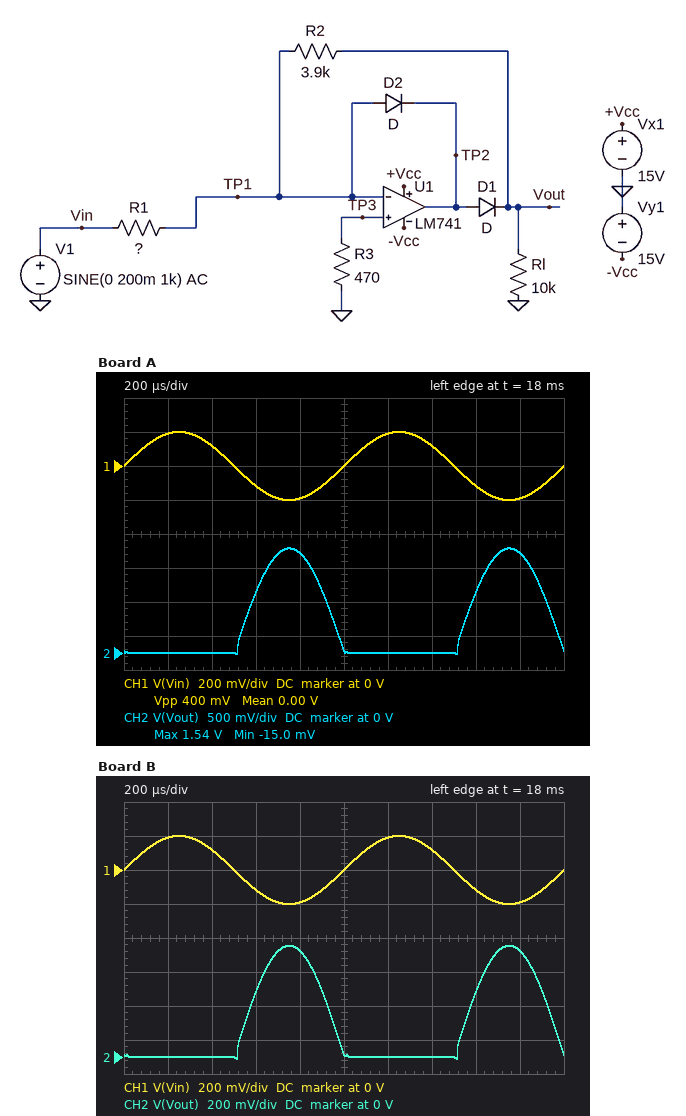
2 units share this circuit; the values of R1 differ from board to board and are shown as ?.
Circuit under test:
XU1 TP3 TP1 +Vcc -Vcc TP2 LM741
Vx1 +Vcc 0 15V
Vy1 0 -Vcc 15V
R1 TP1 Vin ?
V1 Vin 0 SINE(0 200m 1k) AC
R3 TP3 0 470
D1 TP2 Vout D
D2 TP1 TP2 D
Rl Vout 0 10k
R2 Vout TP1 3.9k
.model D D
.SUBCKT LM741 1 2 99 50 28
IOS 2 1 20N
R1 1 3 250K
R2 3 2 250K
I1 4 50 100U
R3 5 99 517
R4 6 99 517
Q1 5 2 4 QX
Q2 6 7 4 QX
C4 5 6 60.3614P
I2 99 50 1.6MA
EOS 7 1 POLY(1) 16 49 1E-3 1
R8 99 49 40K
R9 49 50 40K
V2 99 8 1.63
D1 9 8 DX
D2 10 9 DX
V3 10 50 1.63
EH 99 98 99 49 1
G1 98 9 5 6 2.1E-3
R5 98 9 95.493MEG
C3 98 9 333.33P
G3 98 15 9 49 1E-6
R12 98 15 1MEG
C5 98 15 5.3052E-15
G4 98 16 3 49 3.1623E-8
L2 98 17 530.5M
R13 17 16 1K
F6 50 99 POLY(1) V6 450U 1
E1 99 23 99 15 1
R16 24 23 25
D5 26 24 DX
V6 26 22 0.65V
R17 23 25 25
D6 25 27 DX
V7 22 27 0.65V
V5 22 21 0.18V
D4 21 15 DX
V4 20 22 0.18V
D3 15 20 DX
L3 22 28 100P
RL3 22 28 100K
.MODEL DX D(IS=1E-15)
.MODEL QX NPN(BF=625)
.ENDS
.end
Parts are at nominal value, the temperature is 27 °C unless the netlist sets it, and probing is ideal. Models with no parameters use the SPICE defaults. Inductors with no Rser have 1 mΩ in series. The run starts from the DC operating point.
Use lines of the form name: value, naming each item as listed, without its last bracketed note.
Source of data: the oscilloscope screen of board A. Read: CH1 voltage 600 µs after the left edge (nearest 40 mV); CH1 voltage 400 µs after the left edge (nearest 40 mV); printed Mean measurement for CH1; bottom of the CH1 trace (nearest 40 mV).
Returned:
CH1 voltage 600 µs after the left edge: -120 mV
CH1 voltage 400 µs after the left edge: 120 mV
printed Mean measurement for CH1: 0.00 V
bottom of the CH1 trace: -200 mV
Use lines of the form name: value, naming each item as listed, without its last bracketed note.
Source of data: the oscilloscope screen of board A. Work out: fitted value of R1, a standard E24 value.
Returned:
fitted value of R1, a standard E24 value: 510 Ω
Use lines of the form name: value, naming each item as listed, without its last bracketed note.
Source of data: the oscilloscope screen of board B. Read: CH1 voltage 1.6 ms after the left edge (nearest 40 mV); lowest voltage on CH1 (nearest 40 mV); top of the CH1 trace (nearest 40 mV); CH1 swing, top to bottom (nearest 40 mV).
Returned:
CH1 voltage 1.6 ms after the left edge: -120 mV
lowest voltage on CH1: -200 mV
top of the CH1 trace: 200 mV
CH1 swing, top to bottom: 400 mV
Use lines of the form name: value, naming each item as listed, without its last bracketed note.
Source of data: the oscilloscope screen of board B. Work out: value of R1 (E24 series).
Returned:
value of R1: 1.2 kΩ
